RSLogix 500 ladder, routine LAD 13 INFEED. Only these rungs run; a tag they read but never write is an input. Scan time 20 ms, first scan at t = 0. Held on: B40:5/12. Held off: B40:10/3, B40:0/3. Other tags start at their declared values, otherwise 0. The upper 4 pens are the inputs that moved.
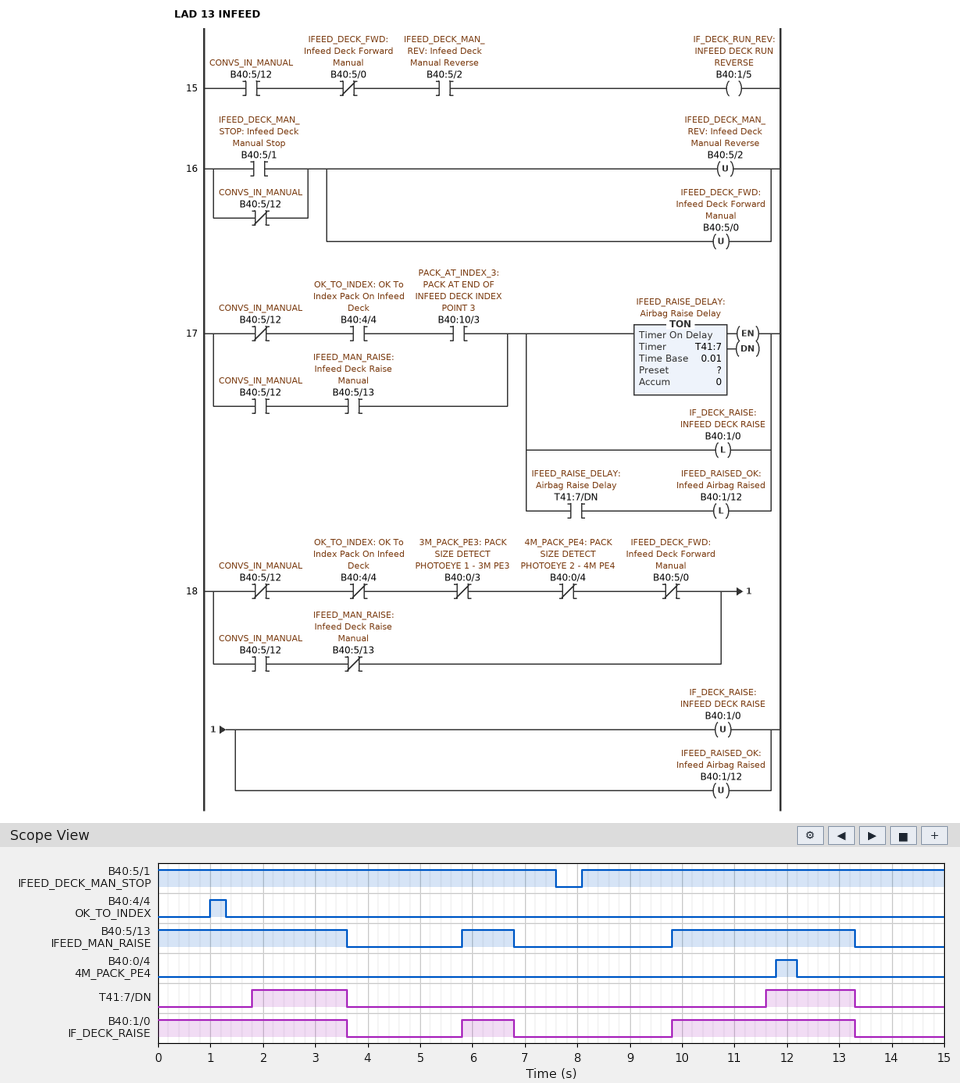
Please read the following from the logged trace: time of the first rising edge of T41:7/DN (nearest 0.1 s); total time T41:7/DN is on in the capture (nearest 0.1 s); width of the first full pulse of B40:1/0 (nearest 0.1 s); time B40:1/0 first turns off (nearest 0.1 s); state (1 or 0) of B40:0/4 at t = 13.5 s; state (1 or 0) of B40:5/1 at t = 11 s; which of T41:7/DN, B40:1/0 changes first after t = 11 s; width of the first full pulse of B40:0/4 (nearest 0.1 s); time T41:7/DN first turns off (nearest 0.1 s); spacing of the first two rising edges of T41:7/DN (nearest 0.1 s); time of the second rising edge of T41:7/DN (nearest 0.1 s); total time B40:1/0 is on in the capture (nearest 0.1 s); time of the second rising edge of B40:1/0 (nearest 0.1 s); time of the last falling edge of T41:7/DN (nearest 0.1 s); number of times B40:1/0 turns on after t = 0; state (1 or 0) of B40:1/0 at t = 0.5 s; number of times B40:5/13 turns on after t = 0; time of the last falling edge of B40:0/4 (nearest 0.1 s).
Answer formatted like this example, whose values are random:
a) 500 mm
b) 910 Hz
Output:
a) 1.8 s
b) 3.5 s
c) 1.0 s
d) 3.6 s
e) 0
f) 1
g) T41:7/DN
h) 0.4 s
i) 3.6 s
j) 9.8 s
k) 11.6 s
l) 8.1 s
m) 9.8 s
n) 13.3 s
o) 2
p) 1
q) 2
r) 12.2 s
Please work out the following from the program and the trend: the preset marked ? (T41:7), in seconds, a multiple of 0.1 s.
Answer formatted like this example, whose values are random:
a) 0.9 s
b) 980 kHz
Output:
a) 1.8 s
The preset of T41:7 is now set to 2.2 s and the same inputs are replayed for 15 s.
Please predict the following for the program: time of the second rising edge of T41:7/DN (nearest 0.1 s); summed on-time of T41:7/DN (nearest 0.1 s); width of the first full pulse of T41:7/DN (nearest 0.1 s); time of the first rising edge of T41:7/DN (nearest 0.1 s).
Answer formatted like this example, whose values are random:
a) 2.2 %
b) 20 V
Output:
a) 12.0 s
b) 2.7 s
c) 1.4 s
d) 2.2 s
